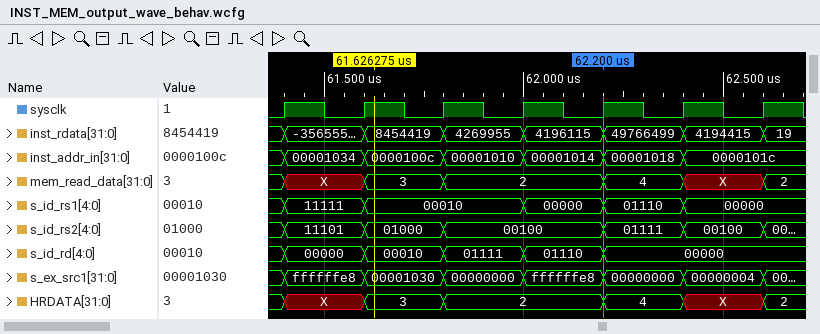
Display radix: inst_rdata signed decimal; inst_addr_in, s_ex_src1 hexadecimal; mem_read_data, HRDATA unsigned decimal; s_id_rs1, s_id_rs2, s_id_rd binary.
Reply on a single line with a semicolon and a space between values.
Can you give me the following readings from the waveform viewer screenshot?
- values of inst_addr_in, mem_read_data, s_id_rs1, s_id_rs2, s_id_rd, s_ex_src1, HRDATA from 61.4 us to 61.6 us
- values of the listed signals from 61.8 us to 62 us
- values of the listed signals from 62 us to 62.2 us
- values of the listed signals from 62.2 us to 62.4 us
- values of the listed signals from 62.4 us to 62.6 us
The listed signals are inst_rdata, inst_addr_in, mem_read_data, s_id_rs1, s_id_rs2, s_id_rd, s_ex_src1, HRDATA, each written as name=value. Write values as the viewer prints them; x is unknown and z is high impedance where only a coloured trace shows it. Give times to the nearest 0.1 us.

inst_addr_in=00001034, mem_read_data=X, s_id_rs1=11111, s_id_rs2=11101, s_id_rd=00000, s_ex_src1=ffffffe8, HRDATA=X; inst_rdata=4269955, inst_addr_in=00001010, mem_read_data=2, s_id_rs1=00010, s_id_rs2=00100, s_id_rd=01111, s_ex_src1=00000000, HRDATA=2; inst_rdata=4196115, inst_addr_in=00001014, mem_read_data=2, s_id_rs1=00000, s_id_rs2=00100, s_id_rd=01110, s_ex_src1=ffffffe8, HRDATA=2; inst_rdata=49766499, inst_addr_in=00001018, mem_read_data=4, s_id_rs1=01110, s_id_rs2=01111, s_id_rd=00000, s_ex_src1=00000000, HRDATA=4; inst_rdata=4194415, inst_addr_in=0000101c, mem_read_data=X, s_id_rs1=00000, s_id_rs2=00100, s_id_rd=00000, s_ex_src1=00000004, HRDATA=X
